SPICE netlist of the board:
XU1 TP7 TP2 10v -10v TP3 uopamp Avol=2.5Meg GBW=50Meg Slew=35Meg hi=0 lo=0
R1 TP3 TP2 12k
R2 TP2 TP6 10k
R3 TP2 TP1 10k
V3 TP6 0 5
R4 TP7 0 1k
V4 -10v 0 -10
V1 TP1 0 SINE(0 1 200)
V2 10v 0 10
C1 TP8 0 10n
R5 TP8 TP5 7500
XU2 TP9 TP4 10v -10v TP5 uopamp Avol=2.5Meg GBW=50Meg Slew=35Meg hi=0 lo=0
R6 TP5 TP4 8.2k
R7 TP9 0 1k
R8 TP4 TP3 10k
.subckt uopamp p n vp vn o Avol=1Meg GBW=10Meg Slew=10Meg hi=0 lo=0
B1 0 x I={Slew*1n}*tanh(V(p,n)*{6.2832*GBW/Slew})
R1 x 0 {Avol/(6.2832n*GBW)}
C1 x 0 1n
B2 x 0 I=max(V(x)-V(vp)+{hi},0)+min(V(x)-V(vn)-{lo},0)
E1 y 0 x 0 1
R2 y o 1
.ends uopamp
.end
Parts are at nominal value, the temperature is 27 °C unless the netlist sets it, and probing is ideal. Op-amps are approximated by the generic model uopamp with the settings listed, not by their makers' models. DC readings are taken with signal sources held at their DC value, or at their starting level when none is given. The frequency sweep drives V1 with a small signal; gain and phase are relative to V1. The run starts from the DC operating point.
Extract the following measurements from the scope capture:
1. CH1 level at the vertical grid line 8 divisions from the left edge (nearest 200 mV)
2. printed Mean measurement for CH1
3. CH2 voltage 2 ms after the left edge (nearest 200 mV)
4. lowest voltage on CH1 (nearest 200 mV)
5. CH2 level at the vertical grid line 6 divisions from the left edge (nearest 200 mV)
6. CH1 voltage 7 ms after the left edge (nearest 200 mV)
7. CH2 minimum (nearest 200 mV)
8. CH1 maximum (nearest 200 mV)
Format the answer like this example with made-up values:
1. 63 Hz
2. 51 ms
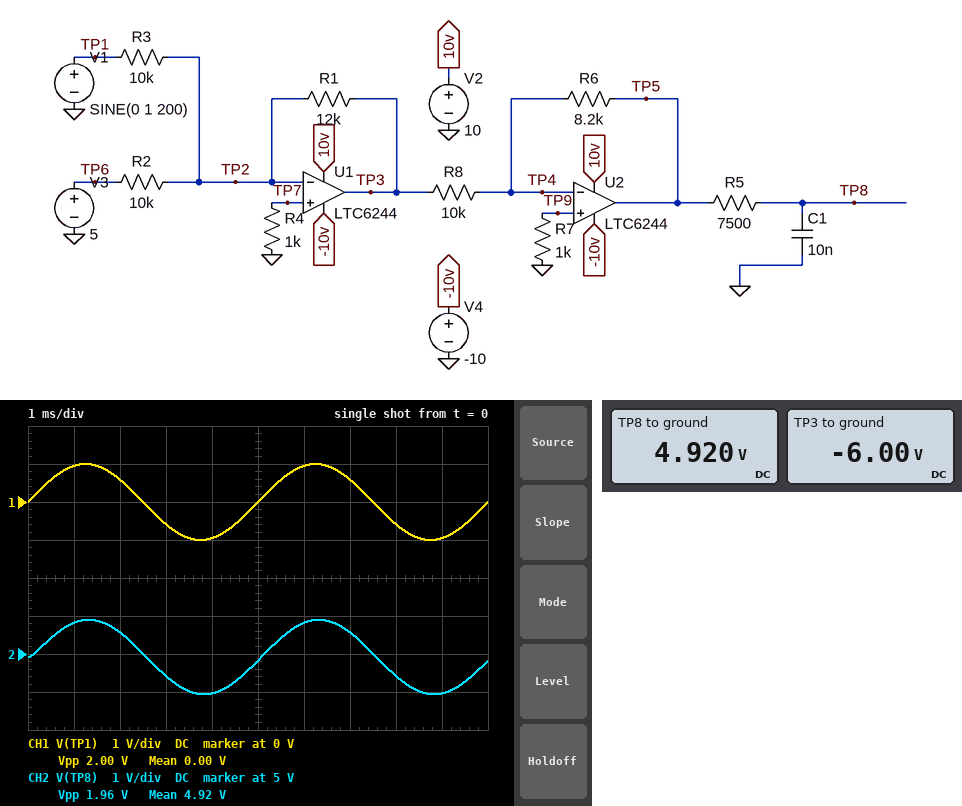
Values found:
1. -600 mV
2. 0.00 V
3. 5.6 V
4. -1.0 V
5. 5.8 V
6. 600 mV
7. 4.0 V
8. 1.0 V
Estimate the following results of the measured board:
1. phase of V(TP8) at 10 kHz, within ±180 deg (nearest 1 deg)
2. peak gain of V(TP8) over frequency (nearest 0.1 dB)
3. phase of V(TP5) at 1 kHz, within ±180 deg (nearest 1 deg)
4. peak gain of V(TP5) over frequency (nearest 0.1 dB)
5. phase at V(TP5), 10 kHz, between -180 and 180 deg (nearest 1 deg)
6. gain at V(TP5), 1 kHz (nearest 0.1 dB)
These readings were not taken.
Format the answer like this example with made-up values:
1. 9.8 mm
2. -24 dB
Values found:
1. -78 deg
2. -0.1 dB
3. 0 deg
4. -0.1 dB
5. 0 deg
6. -0.1 dB
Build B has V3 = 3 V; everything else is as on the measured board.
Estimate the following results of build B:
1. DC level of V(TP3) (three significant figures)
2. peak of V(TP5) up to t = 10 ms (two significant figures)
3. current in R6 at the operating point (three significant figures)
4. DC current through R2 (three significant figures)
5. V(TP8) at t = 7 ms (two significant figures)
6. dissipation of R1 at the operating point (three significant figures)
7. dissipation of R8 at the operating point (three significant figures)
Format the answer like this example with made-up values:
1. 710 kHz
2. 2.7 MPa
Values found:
1. -3.60 V
2. 3.9 V
3. 360 µA
4. 300 µA
5. 3.6 V
6. 1.08 mW
7. 1.30 mW
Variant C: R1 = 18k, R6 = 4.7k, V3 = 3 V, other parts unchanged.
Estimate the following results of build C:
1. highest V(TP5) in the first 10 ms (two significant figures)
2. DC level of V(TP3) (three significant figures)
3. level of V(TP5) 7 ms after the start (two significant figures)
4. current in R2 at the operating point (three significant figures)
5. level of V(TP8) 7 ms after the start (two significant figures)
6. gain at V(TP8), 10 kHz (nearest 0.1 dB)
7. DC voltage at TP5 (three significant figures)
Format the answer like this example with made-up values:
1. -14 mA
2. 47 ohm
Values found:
1. 3.4 V
2. -5.40 V
3. 3.0 V
4. 300 µA
5. 3.1 V
6. -15.1 dB
7. 2.54 V
